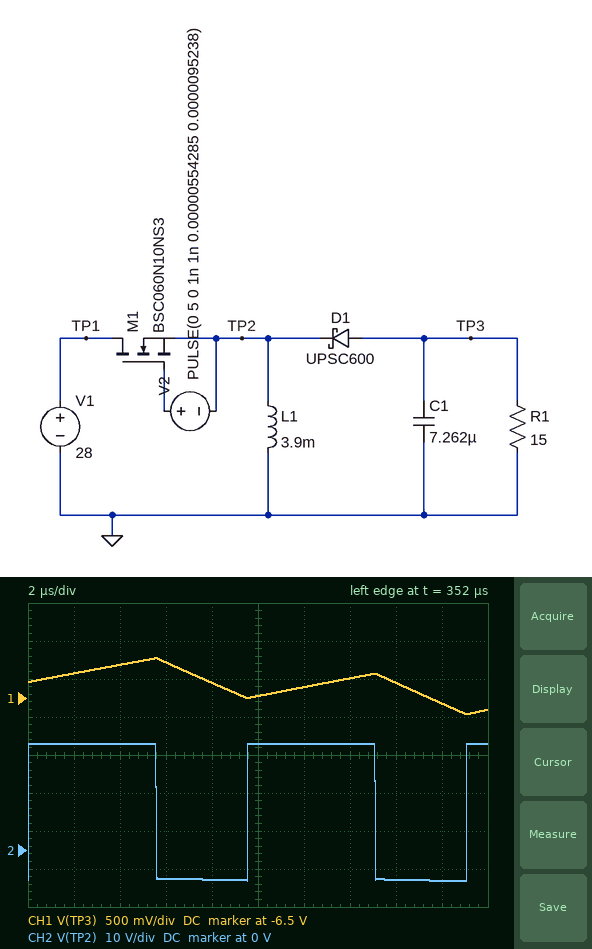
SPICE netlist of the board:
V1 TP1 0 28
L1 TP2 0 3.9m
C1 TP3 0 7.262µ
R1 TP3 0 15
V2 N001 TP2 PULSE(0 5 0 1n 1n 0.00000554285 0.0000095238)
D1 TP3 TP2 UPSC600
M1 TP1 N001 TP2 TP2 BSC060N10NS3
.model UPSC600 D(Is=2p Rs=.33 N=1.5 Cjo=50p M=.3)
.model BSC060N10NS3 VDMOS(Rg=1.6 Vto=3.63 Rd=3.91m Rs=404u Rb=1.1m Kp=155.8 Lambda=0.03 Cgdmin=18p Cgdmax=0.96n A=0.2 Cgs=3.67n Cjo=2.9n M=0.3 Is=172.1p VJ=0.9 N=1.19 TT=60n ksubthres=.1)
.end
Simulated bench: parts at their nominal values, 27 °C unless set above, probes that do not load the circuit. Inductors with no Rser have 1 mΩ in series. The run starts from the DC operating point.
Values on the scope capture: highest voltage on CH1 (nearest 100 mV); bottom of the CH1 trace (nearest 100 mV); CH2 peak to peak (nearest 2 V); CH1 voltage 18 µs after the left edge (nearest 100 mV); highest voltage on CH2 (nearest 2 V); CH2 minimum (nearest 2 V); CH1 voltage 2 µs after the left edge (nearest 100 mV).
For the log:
-6.0 V
-6.7 V
36 V
-6.6 V
28 V
-8 V
-6.2 V
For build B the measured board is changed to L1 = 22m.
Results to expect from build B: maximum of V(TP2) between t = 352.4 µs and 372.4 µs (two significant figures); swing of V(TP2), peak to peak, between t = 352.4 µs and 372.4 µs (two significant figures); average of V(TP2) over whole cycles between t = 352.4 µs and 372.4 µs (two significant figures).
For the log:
28 V
30 V
16 V
